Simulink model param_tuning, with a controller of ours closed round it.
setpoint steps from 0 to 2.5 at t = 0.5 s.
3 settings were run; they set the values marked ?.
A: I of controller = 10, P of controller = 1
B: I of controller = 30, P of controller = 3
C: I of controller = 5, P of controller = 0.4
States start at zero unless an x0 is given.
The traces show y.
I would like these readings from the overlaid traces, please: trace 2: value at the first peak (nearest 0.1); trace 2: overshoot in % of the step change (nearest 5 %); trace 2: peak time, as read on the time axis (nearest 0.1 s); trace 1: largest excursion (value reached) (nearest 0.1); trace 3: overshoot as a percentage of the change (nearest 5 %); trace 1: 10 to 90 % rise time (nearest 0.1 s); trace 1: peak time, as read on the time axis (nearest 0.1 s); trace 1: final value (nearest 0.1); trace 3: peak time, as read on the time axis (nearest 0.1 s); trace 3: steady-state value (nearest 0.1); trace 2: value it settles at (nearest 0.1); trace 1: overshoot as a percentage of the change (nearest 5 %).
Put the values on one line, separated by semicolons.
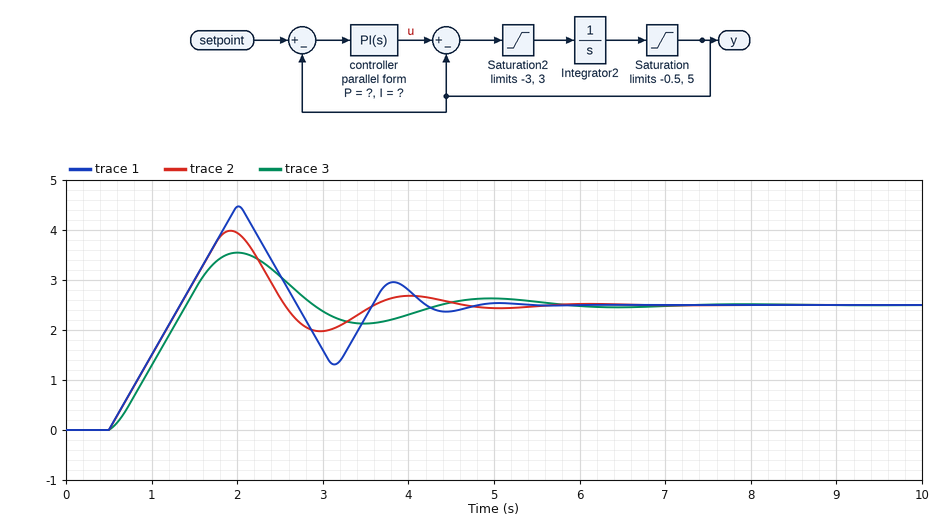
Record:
4.0; 60 %; 1.9 s; 4.5; 40 %; 0.7 s; 2.0 s; 2.5; 2.0 s; 2.5; 2.5; 80 %
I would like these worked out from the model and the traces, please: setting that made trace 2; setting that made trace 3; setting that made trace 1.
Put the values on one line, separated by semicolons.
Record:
A; C; B
